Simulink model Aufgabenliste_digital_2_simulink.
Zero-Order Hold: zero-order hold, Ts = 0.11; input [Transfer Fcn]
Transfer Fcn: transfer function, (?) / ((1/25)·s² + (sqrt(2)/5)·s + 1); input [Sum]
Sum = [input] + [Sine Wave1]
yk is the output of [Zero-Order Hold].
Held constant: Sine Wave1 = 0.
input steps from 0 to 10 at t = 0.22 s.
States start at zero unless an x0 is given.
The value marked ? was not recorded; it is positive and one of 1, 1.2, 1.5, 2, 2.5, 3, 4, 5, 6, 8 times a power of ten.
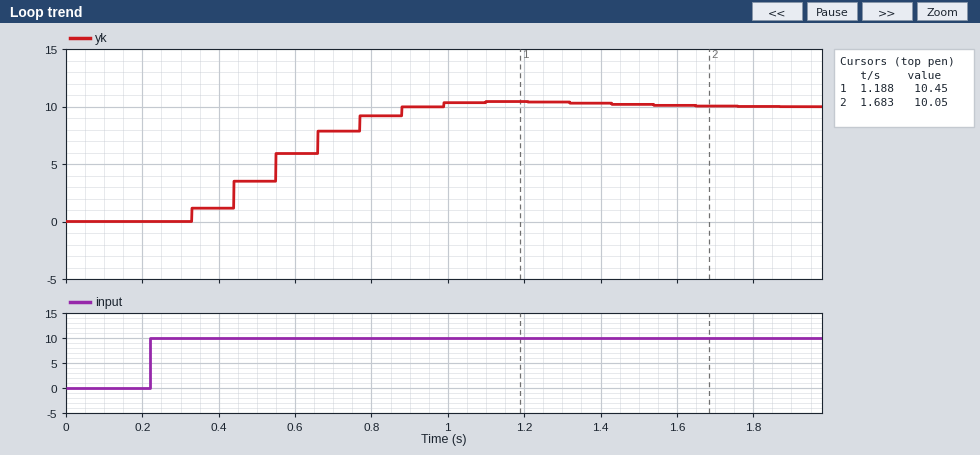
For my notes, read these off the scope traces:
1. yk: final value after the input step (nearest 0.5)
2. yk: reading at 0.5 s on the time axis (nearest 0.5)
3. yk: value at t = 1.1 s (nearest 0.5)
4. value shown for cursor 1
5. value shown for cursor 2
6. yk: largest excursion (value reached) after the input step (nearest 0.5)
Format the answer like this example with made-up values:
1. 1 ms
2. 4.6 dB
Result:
1. 10.0
2. 3.5
3. 10.5
4. 10.45
5. 10.05
6. 10.5
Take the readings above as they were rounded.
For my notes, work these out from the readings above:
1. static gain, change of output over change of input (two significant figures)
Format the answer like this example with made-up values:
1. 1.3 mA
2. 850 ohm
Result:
1. 1.0
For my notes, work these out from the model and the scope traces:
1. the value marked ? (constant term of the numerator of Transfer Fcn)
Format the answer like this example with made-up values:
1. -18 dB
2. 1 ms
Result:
1. 1
